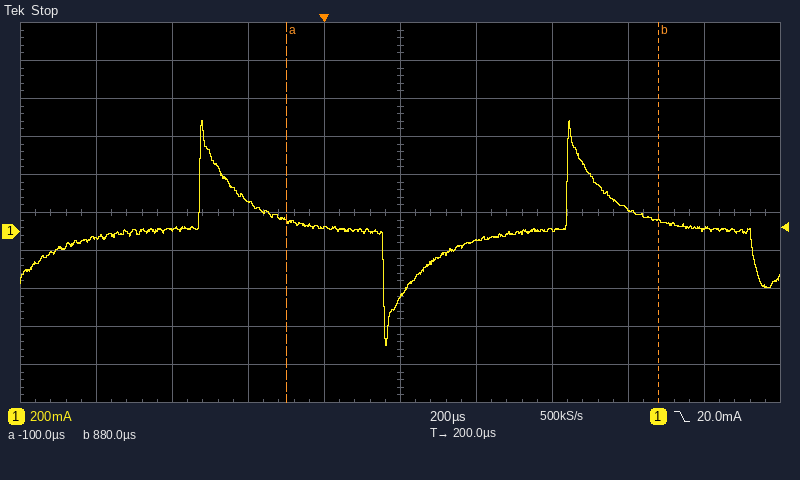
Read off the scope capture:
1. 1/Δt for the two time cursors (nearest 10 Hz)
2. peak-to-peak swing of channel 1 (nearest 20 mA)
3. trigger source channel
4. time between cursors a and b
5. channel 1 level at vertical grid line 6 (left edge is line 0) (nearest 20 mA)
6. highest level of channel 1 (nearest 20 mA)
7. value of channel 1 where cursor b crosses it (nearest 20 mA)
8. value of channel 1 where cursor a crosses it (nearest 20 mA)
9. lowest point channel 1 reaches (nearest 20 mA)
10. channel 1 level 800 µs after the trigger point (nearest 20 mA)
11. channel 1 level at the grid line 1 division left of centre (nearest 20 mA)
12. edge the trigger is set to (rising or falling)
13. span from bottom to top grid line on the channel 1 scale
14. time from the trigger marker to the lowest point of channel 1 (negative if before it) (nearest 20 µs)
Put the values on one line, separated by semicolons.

1.02 kHz; 1.18 A; channel 1; 980 µs; -40 mA; 580 mA; 60 mA; 60 mA; -600 mA; 120 mA; 20 mA; falling; 2 A; +160 µs
